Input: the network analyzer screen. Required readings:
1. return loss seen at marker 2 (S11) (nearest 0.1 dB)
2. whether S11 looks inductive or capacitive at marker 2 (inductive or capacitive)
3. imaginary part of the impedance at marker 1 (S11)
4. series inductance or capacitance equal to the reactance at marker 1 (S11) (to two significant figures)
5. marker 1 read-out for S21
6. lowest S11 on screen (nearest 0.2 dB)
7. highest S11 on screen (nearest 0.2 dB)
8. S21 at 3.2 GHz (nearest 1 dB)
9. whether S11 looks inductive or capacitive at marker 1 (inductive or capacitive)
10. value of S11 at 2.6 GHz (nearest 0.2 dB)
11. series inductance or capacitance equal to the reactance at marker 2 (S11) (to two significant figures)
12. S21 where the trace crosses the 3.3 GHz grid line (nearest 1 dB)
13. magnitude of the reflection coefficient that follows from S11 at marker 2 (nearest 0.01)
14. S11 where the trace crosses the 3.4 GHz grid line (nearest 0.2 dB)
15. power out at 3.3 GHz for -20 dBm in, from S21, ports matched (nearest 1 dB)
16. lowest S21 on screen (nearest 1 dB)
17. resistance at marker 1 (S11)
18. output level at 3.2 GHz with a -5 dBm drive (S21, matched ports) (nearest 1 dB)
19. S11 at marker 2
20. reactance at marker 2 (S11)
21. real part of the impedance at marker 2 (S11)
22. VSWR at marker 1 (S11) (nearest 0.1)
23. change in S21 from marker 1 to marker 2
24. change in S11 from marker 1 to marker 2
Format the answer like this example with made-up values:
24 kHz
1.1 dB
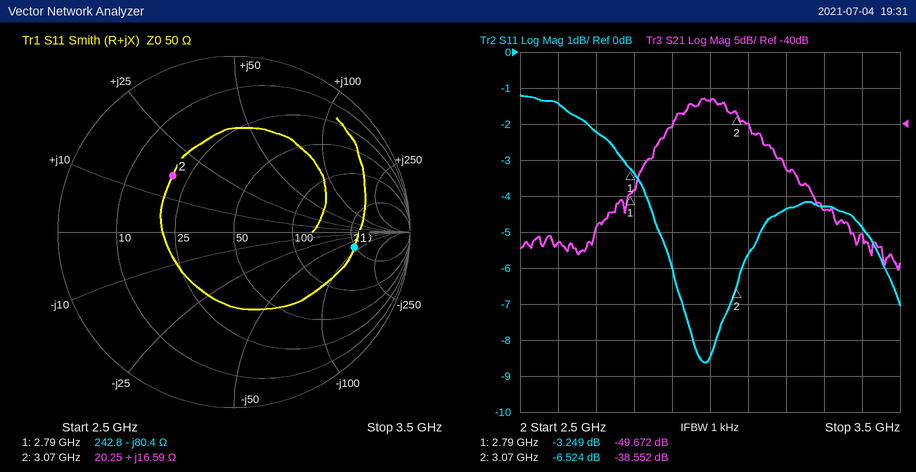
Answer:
6.5 dB
inductive
-80.4 Ω
710 fF
-49.672 dB
-8.6 dB
-1.2 dB
-46 dB
capacitive
-1.4 dB
860 pH
-52 dB
0.47
-4.8 dB
-72 dBm
-60 dB
242.8 Ω
-51 dBm
-6.524 dB
+16.59 Ω
20.25 Ω
5.4
11.120 dB
-3.275 dB
